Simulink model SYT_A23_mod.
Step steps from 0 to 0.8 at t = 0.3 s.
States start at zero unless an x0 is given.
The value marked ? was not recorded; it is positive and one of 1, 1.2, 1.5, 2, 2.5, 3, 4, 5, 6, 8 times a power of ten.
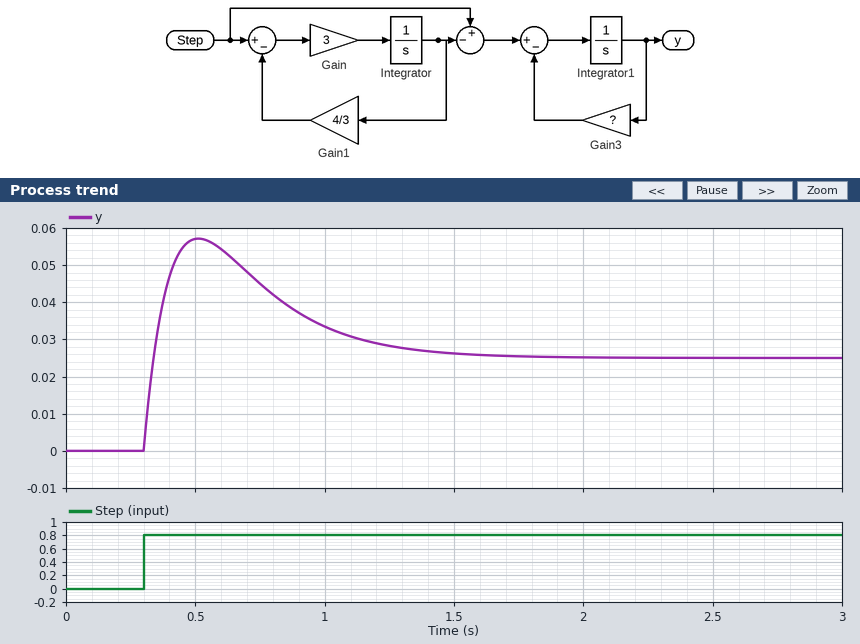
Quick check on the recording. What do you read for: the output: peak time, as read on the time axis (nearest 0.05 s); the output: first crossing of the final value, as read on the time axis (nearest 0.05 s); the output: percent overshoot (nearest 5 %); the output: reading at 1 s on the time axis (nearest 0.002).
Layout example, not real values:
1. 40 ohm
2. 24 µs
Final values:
1. 0.50 s
2. 0.35 s
3. 130 %
4. 0.034
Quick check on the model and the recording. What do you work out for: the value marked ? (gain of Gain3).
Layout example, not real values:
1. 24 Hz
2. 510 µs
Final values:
1. 8
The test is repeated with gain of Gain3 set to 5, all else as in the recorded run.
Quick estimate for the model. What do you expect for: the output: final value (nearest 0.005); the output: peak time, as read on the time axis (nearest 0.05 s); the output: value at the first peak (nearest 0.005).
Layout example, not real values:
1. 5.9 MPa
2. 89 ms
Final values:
1. 0.040
2. 0.60 s
3. 0.080
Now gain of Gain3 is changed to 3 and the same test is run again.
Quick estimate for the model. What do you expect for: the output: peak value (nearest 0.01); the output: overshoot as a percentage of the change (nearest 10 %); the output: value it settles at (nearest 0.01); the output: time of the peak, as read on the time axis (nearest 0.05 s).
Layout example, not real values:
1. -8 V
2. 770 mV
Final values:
1. 0.11
2. 60 %
3. 0.07
4. 0.70 s
